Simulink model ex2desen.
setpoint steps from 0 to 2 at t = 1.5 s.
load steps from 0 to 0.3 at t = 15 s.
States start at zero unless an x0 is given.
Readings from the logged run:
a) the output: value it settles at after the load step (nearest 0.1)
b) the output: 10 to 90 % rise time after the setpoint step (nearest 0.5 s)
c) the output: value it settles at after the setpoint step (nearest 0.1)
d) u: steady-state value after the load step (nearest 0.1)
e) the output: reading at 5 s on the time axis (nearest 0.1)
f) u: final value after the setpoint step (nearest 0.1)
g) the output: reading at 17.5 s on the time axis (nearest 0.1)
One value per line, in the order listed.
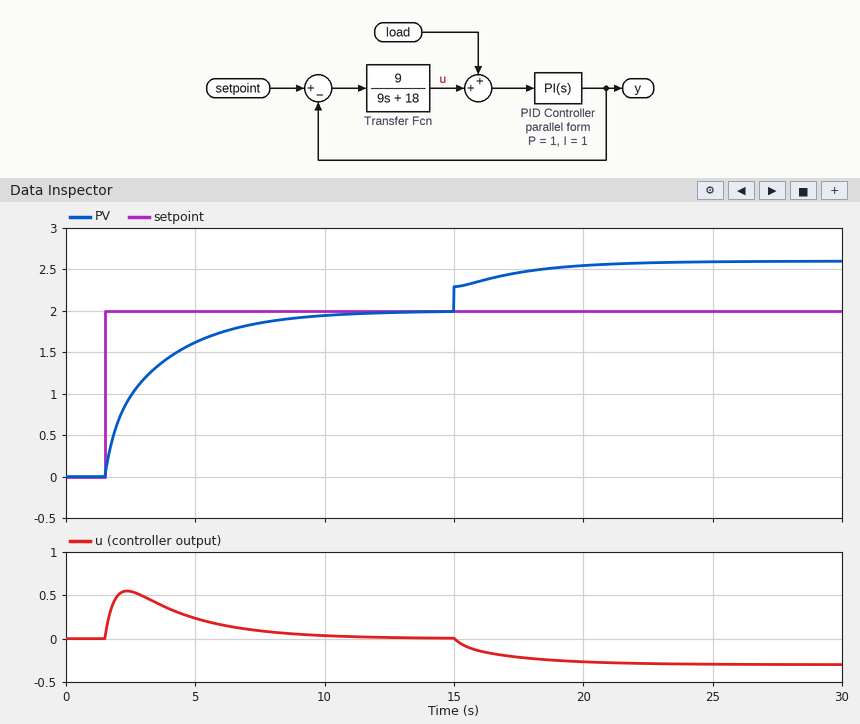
2.6
5.0 s
2.0
-0.3
1.6
0.0
2.5
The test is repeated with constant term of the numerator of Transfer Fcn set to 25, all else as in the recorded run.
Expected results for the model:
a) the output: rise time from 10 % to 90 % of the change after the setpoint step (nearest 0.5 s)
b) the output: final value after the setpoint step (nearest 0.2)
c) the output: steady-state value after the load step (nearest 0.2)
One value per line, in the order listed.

2.0 s
2.0
2.2
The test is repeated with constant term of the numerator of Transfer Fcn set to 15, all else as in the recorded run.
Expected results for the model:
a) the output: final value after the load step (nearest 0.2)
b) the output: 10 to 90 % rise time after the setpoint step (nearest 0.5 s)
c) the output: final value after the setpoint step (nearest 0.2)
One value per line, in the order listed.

2.4
3.0 s
2.0
